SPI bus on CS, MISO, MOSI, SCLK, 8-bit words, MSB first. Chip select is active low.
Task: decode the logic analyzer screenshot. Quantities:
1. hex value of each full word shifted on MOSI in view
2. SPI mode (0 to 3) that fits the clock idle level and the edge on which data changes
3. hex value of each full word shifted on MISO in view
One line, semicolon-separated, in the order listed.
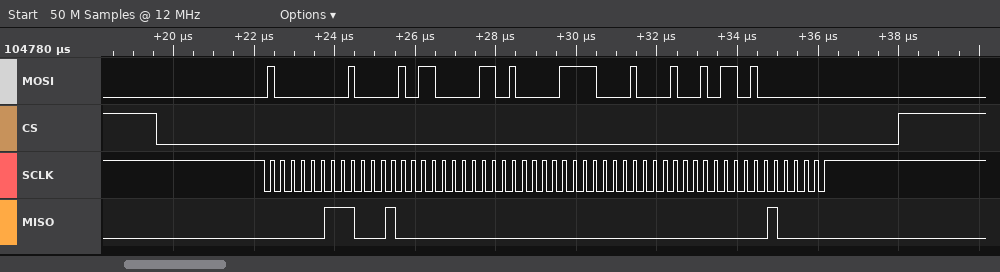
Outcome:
80, 85, 86, 87, 88, 96, 80; 3; 03, 88, 00, 00, 00, 00, 20
